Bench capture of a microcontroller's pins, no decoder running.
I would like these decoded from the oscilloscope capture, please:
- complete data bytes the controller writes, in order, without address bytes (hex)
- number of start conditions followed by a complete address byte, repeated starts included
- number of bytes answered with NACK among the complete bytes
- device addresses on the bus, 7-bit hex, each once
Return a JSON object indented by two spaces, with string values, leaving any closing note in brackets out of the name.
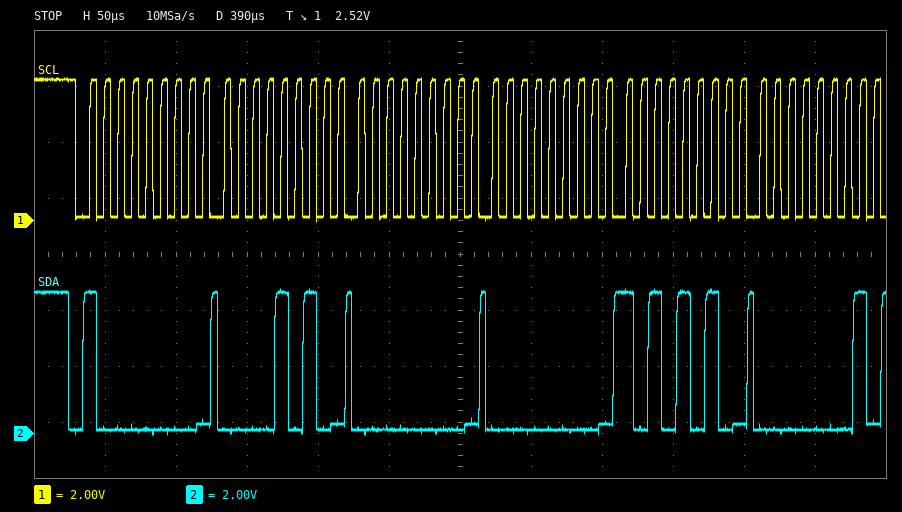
{
  "complete data bytes the controller writes, in order, without address bytes": "0A 00 00 AA 01",
  "number of start conditions followed by a complete address byte, repeated starts included": "1",
  "number of bytes answered with NACK among the complete bytes": "0",
  "device addresses on the bus, 7-bit hex, each once": "0x40"
}
